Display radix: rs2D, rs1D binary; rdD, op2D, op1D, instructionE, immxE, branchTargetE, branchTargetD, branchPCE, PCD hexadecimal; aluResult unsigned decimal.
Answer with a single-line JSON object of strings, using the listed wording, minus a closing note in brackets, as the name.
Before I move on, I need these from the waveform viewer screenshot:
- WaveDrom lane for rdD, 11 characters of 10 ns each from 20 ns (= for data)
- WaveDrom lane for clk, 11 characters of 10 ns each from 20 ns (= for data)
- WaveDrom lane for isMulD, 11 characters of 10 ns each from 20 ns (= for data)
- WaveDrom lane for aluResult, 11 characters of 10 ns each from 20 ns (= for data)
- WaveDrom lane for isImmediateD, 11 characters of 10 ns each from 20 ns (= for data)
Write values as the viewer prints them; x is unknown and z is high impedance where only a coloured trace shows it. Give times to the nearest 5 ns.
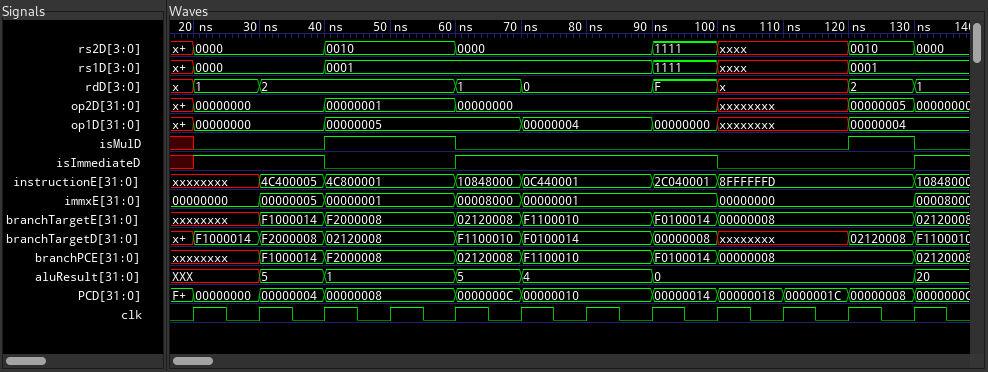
{"WaveDrom lane for rdD, 11 characters of 10 ns each from 20 ns": "{name: 'rdD', wave: '==..==.=x.=', data: '1 2 1 0 F 2'}", "WaveDrom lane for clk, 11 characters of 10 ns each from 20 ns": "{name: 'clk', wave: 'p..........'}", "WaveDrom lane for isMulD, 11 characters of 10 ns each from 20 ns": "{name: 'isMulD', wave: '0.1.0.....1'}", "WaveDrom lane for aluResult, 11 characters of 10 ns each from 20 ns": "{name: 'aluResult', wave: 'x==.==.=...', data: '5 1 5 4 0'}", "WaveDrom lane for isImmediateD, 11 characters of 10 ns each from 20 ns": "{name: 'isImmediateD', wave: '1.0.1...0..'}"}
